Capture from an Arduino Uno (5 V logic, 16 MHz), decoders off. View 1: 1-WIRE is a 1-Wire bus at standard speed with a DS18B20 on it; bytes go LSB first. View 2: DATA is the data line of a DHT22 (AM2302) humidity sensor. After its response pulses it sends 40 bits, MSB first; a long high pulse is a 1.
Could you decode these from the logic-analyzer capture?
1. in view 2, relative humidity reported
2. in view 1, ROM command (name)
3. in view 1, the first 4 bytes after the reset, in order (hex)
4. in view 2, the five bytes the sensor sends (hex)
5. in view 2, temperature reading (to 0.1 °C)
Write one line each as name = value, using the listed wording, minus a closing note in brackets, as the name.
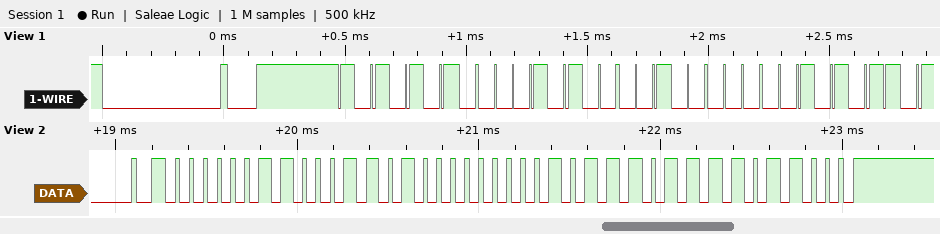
in view 2, relative humidity reported = 79.4 %
in view 1, ROM command = Match ROM
in view 1, the first 4 bytes after the reset, in order = 55 28 04 D4
in view 2, the five bytes the sensor sends = 03 1A 00 BB D8
in view 2, temperature reading = 18.7 °C
